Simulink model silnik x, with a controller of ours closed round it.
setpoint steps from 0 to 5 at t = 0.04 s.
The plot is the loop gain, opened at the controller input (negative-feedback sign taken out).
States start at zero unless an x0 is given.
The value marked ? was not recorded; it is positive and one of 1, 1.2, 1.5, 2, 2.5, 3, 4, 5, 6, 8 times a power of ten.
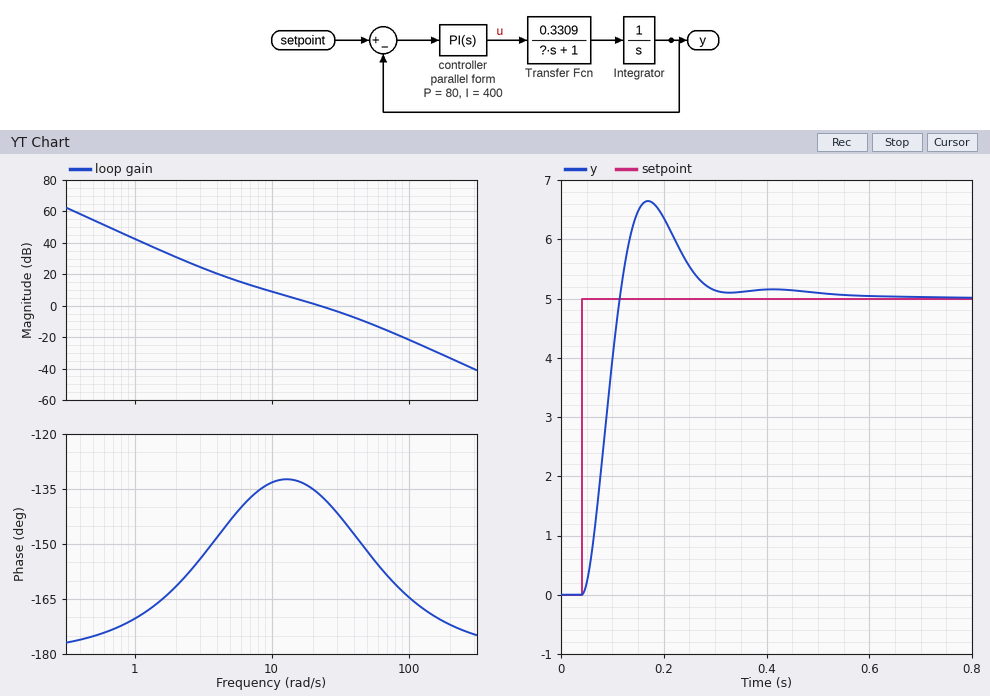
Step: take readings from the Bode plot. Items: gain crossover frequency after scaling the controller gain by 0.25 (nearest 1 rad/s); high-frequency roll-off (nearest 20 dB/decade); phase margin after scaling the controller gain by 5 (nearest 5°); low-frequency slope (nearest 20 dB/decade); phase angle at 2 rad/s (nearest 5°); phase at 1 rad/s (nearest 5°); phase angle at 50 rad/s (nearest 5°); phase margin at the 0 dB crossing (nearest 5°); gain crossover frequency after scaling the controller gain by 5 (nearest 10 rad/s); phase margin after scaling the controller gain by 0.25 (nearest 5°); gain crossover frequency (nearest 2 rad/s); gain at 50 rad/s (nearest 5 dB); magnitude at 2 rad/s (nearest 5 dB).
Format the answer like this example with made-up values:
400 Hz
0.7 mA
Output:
8 rad/s
-40 dB/decade
25°
-40 dB/decade
-160°
-170°
-150°
45°
60 rad/s
45°
22 rad/s
-10 dB
30 dB
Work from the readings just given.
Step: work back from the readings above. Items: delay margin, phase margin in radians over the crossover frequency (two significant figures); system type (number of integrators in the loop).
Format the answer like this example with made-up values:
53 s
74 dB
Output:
0.036 s
2
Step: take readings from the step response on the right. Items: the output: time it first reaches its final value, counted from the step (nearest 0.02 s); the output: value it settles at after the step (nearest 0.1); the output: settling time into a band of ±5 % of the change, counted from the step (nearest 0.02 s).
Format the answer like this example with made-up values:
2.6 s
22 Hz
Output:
0.08 s
5.0
0.24 s
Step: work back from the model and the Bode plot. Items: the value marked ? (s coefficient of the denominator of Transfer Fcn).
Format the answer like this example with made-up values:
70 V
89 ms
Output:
0.03
